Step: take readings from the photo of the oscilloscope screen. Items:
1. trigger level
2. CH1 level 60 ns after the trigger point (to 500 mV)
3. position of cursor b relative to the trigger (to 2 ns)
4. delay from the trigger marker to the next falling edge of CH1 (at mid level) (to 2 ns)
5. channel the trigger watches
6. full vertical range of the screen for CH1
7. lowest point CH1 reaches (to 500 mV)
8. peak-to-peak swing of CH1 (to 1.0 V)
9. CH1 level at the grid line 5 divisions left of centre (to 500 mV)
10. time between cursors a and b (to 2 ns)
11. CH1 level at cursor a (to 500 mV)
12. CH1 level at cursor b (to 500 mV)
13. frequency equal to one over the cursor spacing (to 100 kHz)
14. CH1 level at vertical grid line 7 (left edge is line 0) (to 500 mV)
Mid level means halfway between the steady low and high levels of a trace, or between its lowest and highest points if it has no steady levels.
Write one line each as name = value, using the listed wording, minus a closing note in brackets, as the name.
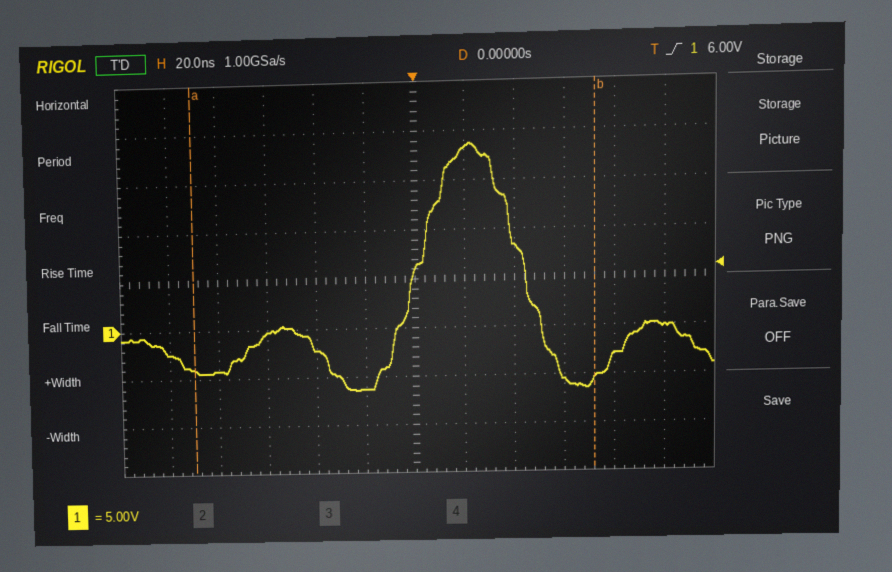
trigger level = 6.00 V
CH1 level 60 ns after the trigger point = -5.5 V
position of cursor b relative to the trigger = +72 ns
delay from the trigger marker to the next falling edge of CH1 (at mid level) = 44 ns
channel the trigger watches = CH1
full vertical range of the screen for CH1 = 40 V
lowest point CH1 reaches = -6.5 V
peak-to-peak swing of CH1 = 25.0 V
CH1 level at the grid line 5 divisions left of centre = -2.5 V
time between cursors a and b = 162 ns
CH1 level at cursor a = -4.0 V
CH1 level at cursor b = -5.5 V
frequency equal to one over the cursor spacing = 6.2 MHz
CH1 level at vertical grid line 7 (left edge is line 0) = 18.5 V
